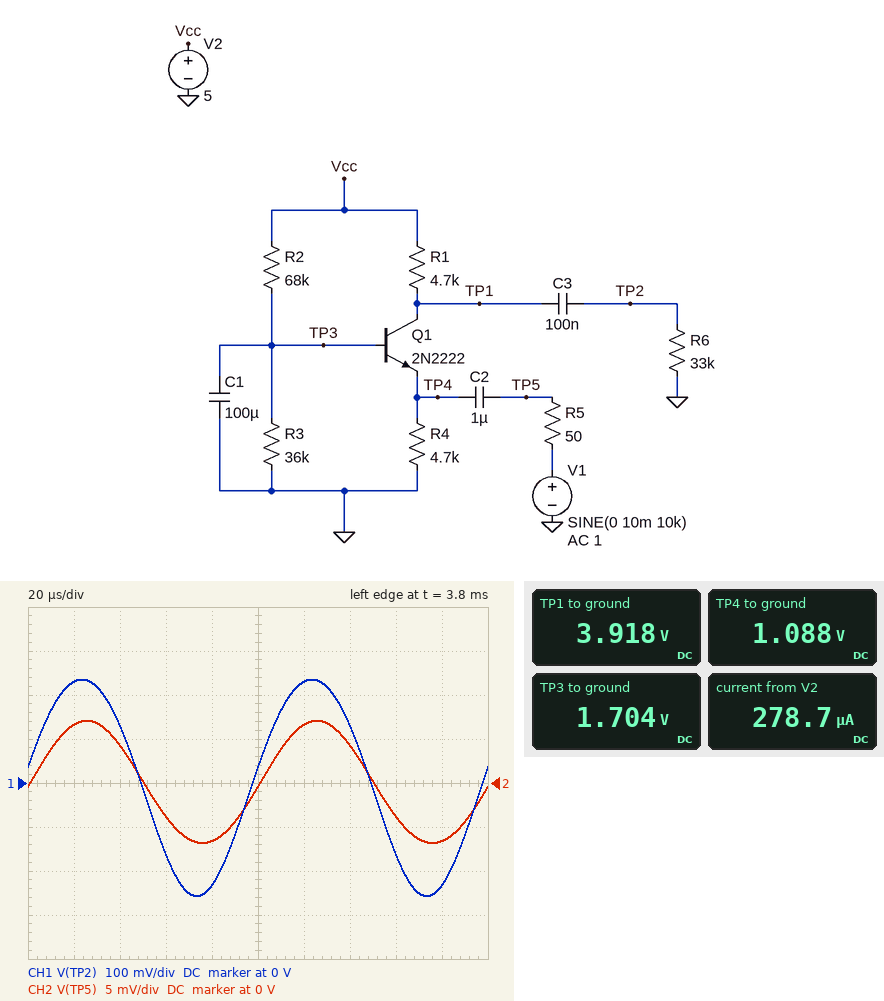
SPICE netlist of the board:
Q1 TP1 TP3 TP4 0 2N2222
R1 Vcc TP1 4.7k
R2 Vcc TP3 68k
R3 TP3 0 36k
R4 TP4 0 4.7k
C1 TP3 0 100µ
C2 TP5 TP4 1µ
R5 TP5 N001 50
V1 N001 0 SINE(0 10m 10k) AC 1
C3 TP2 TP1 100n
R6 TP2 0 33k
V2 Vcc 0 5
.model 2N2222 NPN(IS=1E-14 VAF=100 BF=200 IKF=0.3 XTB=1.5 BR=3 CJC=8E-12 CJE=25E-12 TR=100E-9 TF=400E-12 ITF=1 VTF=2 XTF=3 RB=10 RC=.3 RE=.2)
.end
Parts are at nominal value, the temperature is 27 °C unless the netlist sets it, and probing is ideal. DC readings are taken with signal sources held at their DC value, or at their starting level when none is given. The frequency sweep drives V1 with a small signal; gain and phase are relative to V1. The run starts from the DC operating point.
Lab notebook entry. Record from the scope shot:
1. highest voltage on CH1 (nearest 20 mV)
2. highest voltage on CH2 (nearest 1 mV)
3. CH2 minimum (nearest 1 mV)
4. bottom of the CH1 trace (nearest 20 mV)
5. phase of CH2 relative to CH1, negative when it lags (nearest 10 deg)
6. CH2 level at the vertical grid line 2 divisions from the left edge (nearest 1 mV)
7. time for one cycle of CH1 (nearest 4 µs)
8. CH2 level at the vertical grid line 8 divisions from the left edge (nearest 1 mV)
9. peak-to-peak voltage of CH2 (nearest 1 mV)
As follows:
240 mV
7 mV
-7 mV
-260 mV
-10 deg
4 mV
100 µs
-4 mV
14 mV
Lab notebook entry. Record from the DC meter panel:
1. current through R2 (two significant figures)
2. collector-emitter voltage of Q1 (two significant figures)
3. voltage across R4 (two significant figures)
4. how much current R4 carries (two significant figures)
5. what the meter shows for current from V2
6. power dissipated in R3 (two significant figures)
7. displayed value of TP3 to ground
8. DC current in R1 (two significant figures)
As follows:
48 µA
2.8 V
1.1 V
230 µA
278.7 µA
81 µW
1.704 V
230 µA
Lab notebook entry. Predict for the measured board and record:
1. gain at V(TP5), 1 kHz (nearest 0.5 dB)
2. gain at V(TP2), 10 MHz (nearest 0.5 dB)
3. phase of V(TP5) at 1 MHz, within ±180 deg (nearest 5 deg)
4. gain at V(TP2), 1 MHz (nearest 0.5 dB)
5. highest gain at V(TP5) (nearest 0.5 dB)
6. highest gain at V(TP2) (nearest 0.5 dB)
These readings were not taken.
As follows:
-1.5 dB
23.0 dB
0 deg
28.0 dB
0 dB
28.0 dB
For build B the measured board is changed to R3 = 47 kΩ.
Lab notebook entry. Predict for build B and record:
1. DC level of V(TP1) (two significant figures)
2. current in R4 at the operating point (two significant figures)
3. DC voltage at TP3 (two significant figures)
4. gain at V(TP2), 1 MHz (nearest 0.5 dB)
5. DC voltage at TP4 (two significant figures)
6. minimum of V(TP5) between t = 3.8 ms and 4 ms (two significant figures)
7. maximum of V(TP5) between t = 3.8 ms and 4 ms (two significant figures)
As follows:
3.6 V
290 µA
2.0 V
29.0 dB
1.4 V
-6.3 mV
6.6 mV
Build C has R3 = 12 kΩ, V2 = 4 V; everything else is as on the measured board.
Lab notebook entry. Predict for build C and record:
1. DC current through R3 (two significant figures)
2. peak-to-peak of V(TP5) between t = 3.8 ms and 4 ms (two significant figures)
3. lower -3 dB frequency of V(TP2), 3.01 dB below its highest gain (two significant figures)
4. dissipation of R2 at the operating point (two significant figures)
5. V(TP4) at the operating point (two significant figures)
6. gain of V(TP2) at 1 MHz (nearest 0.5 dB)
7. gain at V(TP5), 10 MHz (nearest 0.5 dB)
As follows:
50 µA
19 mV
120 Hz
170 µW
59 mV
5.5 dB
-0.5 dB
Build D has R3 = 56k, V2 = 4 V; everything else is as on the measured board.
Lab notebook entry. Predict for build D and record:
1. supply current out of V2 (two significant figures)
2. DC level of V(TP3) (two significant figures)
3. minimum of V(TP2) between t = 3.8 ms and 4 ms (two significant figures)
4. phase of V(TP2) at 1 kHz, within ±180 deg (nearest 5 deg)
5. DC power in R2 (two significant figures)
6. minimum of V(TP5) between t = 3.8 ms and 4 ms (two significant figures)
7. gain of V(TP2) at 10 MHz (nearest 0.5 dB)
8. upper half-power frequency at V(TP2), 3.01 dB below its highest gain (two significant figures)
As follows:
280 µA
1.8 V
-270 mV
50 deg
73 µW
-6.7 mV
22.5 dB
6.1 MHz
